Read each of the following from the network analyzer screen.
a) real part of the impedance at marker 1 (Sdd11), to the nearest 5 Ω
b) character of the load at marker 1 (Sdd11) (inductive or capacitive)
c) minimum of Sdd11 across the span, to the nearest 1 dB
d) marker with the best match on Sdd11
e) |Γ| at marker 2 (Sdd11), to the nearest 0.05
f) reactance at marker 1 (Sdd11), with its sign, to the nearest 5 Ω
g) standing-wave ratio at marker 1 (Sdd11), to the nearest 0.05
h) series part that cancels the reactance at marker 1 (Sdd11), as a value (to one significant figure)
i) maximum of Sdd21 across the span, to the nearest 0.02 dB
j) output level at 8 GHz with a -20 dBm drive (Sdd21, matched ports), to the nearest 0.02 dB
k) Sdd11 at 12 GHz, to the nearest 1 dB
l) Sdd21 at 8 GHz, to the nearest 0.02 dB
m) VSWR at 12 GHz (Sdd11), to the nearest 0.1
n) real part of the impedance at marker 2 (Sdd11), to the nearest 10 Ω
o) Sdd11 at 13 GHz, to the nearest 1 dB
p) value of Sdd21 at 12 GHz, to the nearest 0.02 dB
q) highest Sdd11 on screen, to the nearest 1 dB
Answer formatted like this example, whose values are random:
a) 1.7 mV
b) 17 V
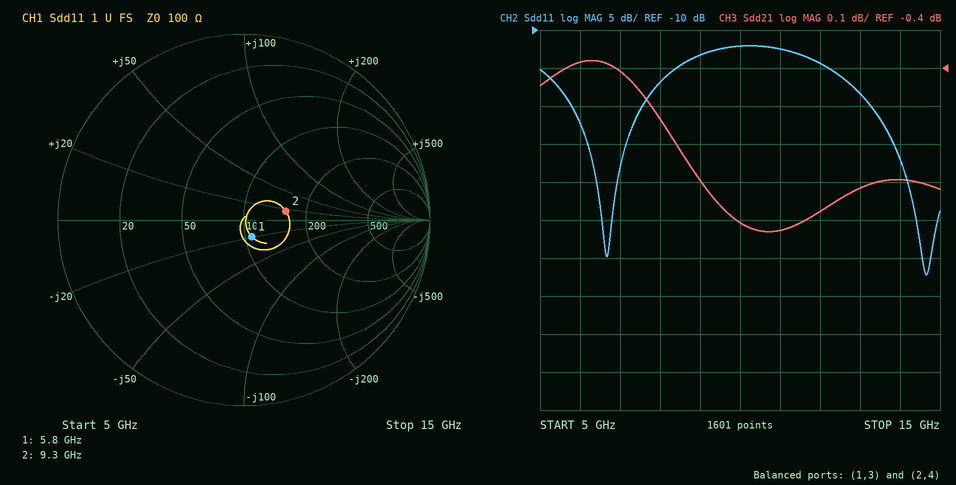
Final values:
a) 105 Ω
b) capacitive
c) -42 dB
d) marker 1
e) 0.25
f) -20 Ω
g) 1.20
h) 500 pH
i) -0.38 dB
j) -20.54 dBm
k) -14 dB
l) -0.54 dB
m) 1.5
n) 160 Ω
o) -18 dB
p) -0.78 dB
q) -12 dB
